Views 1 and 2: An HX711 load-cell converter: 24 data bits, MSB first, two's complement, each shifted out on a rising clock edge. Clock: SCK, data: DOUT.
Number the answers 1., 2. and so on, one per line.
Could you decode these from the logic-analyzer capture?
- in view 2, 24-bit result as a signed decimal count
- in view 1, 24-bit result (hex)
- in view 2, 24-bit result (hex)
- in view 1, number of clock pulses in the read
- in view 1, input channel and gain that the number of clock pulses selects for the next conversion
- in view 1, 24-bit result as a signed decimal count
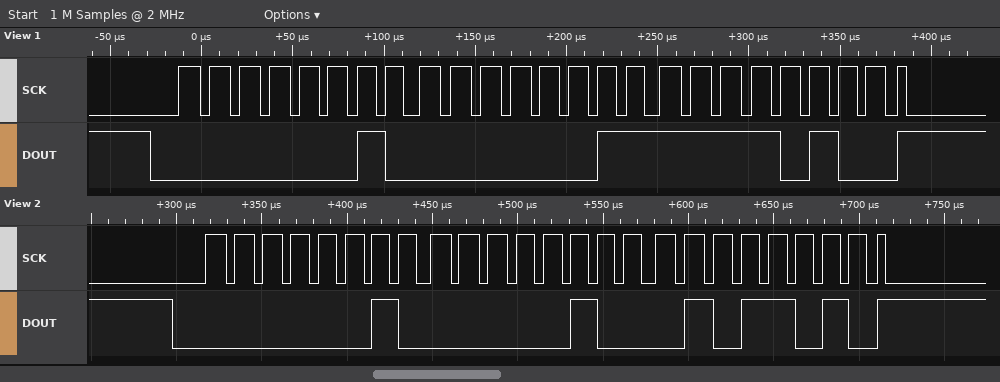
1. 132186
2. 0x0203F4
3. 0x02045A
4. 25
5. channel A, gain 128
6. 132084
